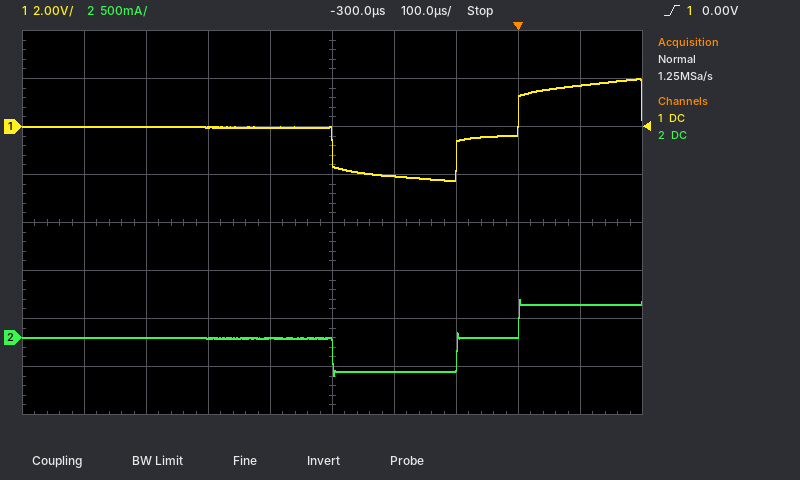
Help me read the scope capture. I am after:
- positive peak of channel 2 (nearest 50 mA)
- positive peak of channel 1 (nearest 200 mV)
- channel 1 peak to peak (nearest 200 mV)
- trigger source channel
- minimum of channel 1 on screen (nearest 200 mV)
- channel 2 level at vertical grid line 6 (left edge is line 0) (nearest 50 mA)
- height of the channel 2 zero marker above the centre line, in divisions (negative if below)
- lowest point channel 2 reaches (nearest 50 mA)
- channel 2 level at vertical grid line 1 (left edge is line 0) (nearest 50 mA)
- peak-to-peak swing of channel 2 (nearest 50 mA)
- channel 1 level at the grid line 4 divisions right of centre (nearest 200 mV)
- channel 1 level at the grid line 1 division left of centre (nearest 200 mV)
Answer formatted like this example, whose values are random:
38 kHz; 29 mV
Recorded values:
400 mA; 2.0 V; 4.2 V; channel 1; -2.2 V; -350 mA; -2.4 div; -400 mA; 0 mA; 800 mA; 1.8 V; 0.0 V
